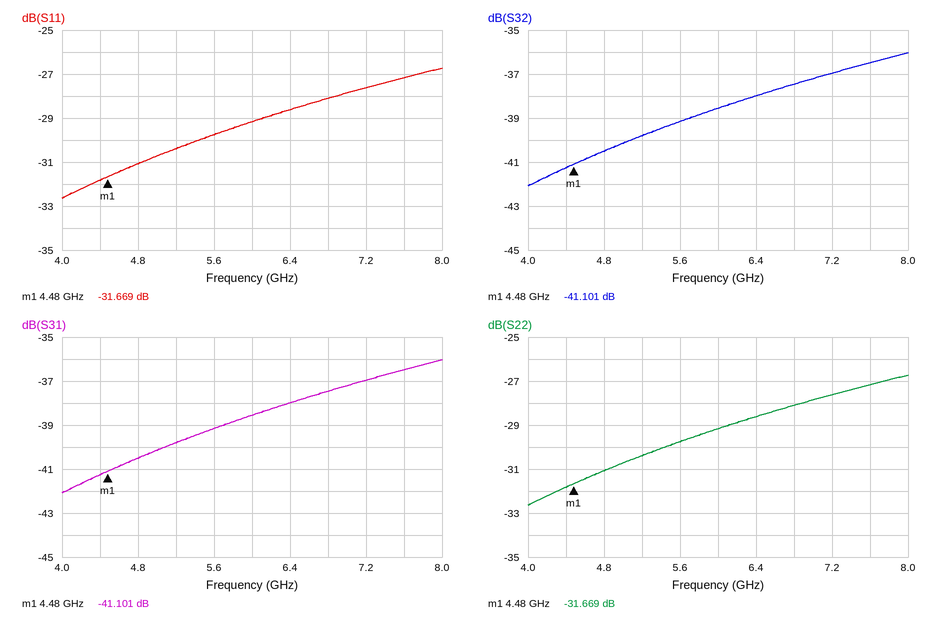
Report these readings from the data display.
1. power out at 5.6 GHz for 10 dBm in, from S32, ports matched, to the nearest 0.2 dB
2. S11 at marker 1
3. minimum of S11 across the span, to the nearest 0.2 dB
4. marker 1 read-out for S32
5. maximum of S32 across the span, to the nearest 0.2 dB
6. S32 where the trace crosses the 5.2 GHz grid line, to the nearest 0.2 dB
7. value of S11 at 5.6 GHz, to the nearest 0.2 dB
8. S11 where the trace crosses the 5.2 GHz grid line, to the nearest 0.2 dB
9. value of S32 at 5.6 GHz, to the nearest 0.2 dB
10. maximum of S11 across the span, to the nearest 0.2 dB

-29.2 dBm
-31.669 dB
-32.6 dB
-41.101 dB
-36.0 dB
-39.8 dB
-29.8 dB
-30.4 dB
-39.2 dB
-26.8 dB
